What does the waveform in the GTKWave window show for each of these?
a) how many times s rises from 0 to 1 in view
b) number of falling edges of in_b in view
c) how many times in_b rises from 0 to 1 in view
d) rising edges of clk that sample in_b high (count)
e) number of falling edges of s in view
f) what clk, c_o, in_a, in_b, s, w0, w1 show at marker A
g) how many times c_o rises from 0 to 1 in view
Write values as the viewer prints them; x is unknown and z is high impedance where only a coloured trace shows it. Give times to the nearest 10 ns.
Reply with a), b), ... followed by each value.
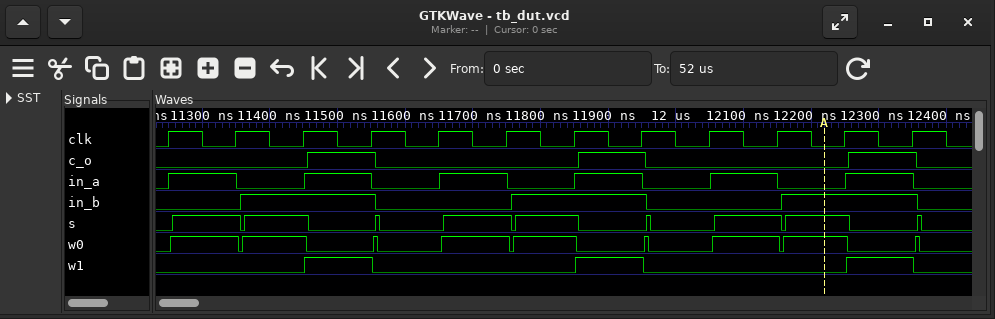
a) 9
b) 3
c) 3
d) 6
e) 9
f) clk=0, c_o=0, in_a=0, in_b=1, s=1, w0=1, w1=0
g) 3
